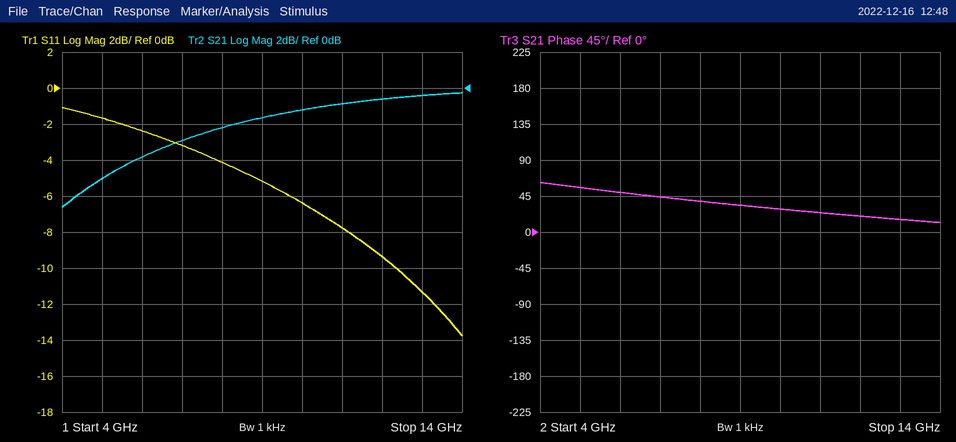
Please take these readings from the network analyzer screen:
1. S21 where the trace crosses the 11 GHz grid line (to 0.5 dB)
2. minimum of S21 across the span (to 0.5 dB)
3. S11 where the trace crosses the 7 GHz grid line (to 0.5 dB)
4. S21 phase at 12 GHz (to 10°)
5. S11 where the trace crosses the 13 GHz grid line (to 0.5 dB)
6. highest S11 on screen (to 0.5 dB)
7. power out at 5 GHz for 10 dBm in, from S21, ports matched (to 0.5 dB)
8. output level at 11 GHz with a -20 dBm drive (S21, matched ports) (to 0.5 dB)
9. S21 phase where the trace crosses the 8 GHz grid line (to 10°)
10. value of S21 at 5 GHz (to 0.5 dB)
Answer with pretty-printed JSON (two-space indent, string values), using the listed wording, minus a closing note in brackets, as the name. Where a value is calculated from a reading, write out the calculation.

{
  "S21 where the trace crosses the 11 GHz grid line": "-1.0 dB",
  "minimum of S21 across the span": "-6.5 dB",
  "S11 where the trace crosses the 7 GHz grid line": "-3.0 dB",
  "S21 phase at 12 GHz": "20°",
  "S11 where the trace crosses the 13 GHz grid line": "-11.5 dB",
  "highest S11 on screen": "-1.0 dB",
  "power out at 5 GHz for 10 dBm in, from S21, ports matched": "10 dBm + (-5.0 dB) = 5.0 dBm",
  "output level at 11 GHz with a -20 dBm drive (S21, matched ports)": "-20 dBm + (-1.0 dB) = -21.0 dBm",
  "S21 phase where the trace crosses the 8 GHz grid line": "40°",
  "value of S21 at 5 GHz": "-5.0 dB"
}
